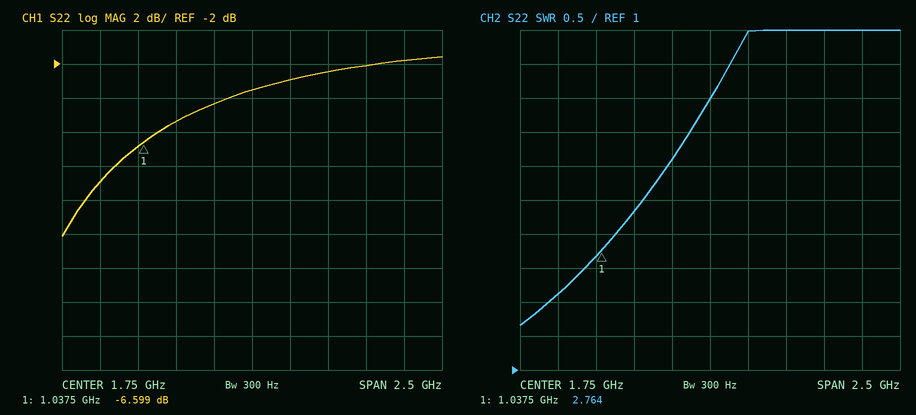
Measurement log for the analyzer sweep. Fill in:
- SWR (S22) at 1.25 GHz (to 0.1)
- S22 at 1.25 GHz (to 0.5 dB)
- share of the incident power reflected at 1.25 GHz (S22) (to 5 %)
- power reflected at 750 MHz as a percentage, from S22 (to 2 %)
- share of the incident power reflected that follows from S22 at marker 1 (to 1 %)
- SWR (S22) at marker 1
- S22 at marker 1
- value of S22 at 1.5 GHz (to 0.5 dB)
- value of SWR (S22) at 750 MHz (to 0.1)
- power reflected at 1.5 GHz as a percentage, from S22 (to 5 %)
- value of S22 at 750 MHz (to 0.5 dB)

3.3
-5.5 dB
30 %
12 %
22 %
2.764
-6.599 dB
-4.5 dB
2.1
35 %
-9.0 dB
